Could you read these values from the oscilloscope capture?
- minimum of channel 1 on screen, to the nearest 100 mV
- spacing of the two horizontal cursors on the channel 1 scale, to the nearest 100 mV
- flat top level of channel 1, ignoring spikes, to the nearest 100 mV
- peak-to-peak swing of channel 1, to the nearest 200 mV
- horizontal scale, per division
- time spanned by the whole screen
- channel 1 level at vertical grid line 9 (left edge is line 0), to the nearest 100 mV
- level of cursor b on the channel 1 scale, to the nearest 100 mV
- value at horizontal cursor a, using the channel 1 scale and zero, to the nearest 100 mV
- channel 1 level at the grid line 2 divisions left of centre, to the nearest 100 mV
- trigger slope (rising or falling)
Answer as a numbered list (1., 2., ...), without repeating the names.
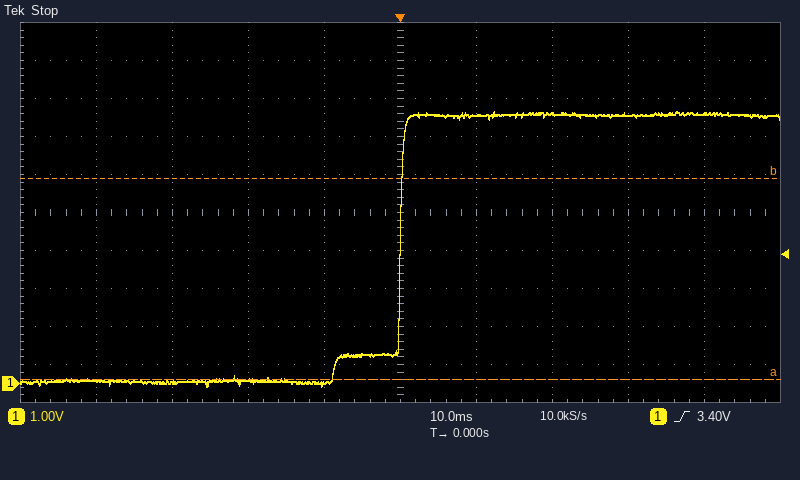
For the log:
1. -100 mV
2. 5.3 V
3. 7.1 V
4. 7.2 V
5. 10 ms
6. 100 ms
7. 7.1 V
8. 5.4 V
9. 100 mV
10. 100 mV
11. rising
